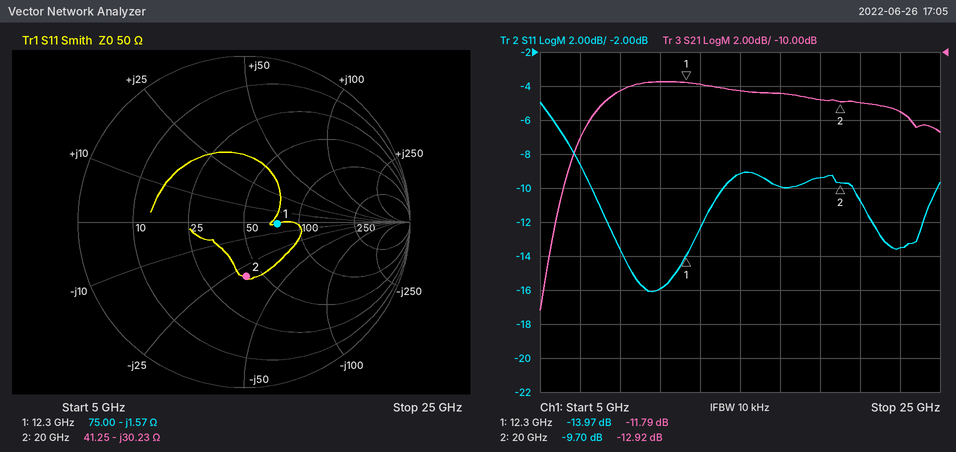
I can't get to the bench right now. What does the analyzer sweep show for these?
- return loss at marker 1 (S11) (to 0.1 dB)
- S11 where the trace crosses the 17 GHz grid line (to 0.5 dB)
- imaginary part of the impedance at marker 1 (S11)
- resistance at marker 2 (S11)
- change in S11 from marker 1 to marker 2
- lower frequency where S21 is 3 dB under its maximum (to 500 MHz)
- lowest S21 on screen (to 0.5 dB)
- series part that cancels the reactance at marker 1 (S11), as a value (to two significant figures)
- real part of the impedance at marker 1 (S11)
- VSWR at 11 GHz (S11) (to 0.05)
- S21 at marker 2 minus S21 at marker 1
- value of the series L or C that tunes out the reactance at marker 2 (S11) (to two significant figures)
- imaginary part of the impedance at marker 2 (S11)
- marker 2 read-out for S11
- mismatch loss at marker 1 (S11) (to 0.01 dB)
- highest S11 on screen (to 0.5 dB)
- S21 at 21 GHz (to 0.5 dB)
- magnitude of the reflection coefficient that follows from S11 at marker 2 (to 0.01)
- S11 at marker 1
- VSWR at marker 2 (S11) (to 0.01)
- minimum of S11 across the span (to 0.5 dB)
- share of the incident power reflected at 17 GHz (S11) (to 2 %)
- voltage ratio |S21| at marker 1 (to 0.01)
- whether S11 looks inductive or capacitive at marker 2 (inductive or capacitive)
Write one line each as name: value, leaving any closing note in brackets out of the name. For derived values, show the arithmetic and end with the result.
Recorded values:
return loss at marker 1 (S11): 14.0 dB
S11 where the trace crosses the 17 GHz grid line: -10.0 dB
imaginary part of the impedance at marker 1: -1.57 Ω
resistance at marker 2: 41.25 Ω
change in S11 from marker 1 to marker 2: -9.7 − (-13.97) = 4.27 dB
lower frequency where S21 is 3 dB under its maximum: 7.0 GHz
lowest S21 on screen: -25.0 dB
series part that cancels the reactance at marker 1 (S11), as a value: L = 1.57 Ω/(2π × 12.3 GHz) ≈ 20 pH
real part of the impedance at marker 1: 75.00 Ω
VSWR at 11 GHz (S11): |Γ| = 10^(-16/20) = 0.1585; VSWR = (1 + 0.1585)/(1 − 0.1585) ≈ 1.38, so 1.40 to the nearest 0.05
S21 at marker 2 minus S21 at marker 1: -12.92 − (-11.79) = -1.13 dB
value of the series L or C that tunes out the reactance at marker 2 (S11): L = 30.23 Ω/(2π × 20 GHz) ≈ 241 pH, so 240 pH to two significant figures
imaginary part of the impedance at marker 2: -30.23 Ω
marker 2 read-out for S11: -9.70 dB
mismatch loss at marker 1 (S11): −10 log10(1 − 10^(-13.97/10)) ≈ 0.18 dB
highest S11 on screen: -5.0 dB
S21 at 21 GHz: -13.0 dB
magnitude of the reflection coefficient that follows from S11 at marker 2: 10^(-9.7/20) ≈ 0.33
S11 at marker 1: -13.97 dB
VSWR at marker 2 (S11): 1.97
minimum of S11 across the span: -16.0 dB
share of the incident power reflected at 17 GHz (S11): 10^(-10/10) ≈ 10 %
voltage ratio |S21| at marker 1: 10^(-11.79/20) ≈ 0.26
whether S11 looks inductive or capacitive at marker 2: capacitive
